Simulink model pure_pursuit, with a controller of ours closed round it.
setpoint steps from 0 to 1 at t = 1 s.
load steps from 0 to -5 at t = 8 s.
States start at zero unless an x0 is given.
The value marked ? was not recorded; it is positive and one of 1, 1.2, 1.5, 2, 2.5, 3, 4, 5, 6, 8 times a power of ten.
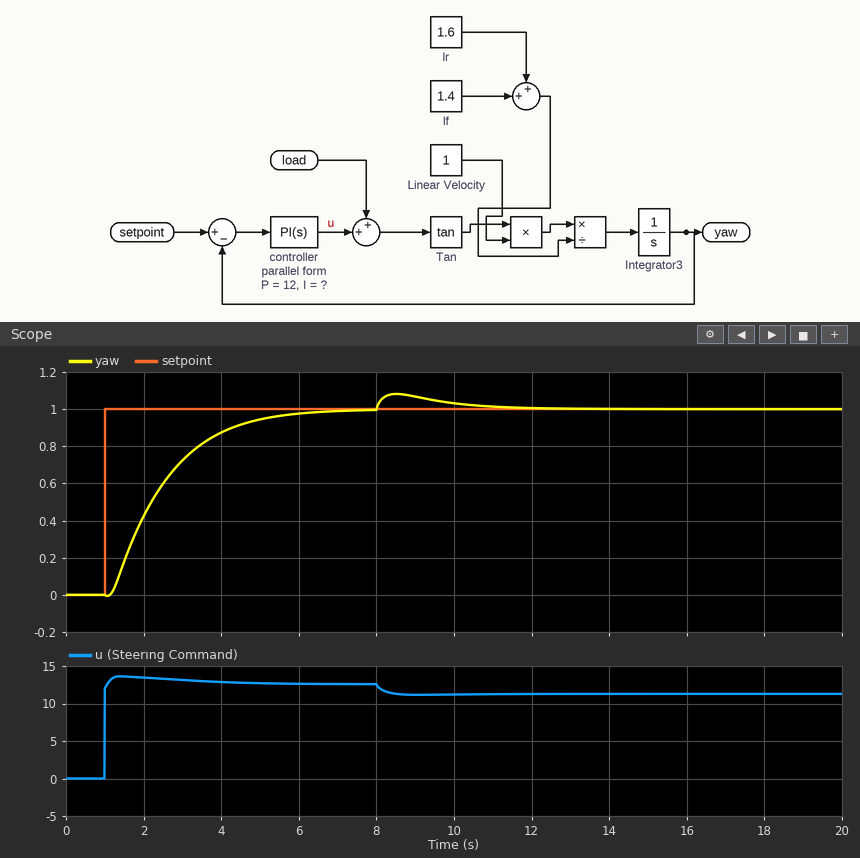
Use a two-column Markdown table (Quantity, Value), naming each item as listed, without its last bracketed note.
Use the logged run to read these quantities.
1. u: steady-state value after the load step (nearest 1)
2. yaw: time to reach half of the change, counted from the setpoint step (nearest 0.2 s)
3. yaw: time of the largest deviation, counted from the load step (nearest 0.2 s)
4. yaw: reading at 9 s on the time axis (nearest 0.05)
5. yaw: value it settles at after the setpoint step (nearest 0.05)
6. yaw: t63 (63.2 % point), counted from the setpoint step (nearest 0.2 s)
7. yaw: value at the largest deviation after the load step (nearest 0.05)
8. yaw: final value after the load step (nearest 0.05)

| Quantity | Value |
|---|---|
| u: steady-state value after the load step | 11 |
| yaw: time to reach half of the change, counted from the setpoint step | 1.2 s |
| yaw: time of the largest deviation, counted from the load step | 0.6 s |
| yaw: reading at 9 s on the time axis | 1.05 |
| yaw: value it settles at after the setpoint step | 1.00 |
| yaw: t63 (63.2 % point), counted from the setpoint step | 1.6 s |
| yaw: value at the largest deviation after the load step | 1.10 |
| yaw: final value after the load step | 1.00 |
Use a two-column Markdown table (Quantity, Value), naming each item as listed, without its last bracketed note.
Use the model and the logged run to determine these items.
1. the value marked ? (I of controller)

| Quantity | Value |
|---|---|
| the value marked ? | 8 |
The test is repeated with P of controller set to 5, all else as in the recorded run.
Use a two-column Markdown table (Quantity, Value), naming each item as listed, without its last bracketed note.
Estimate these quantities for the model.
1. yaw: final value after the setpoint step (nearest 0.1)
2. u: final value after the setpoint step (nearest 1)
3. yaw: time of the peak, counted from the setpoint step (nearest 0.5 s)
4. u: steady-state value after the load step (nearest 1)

| Quantity | Value |
|---|---|
| yaw: final value after the setpoint step | 1.0 |
| u: final value after the setpoint step | 6 |
| yaw: time of the peak, counted from the setpoint step | 2.5 s |
| u: steady-state value after the load step | 5 |
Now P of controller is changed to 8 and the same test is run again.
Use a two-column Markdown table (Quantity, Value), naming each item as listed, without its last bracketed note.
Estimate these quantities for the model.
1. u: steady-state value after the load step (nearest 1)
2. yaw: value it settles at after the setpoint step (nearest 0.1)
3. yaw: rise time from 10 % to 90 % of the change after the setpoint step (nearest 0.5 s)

| Quantity | Value |
|---|---|
| u: steady-state value after the load step | 8 |
| yaw: value it settles at after the setpoint step | 1.0 |
| yaw: rise time from 10 % to 90 % of the change after the setpoint step | 2.0 s |
